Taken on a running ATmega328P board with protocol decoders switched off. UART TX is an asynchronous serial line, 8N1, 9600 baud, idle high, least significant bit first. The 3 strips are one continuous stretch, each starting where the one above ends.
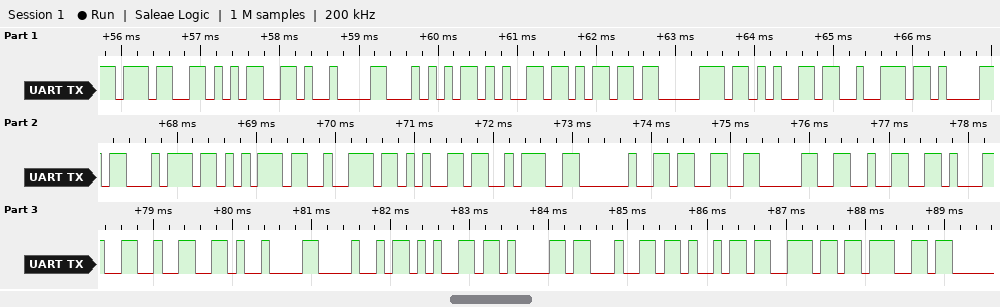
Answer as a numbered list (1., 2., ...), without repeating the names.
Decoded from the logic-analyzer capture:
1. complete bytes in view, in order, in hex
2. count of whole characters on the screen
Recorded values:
1. 37 35 09 54 65 6D 70 65 72 61 74 75 72 65 3A 20 33 30 32 31 32 09 48 65 61 64 69 6E 67
2. 29
